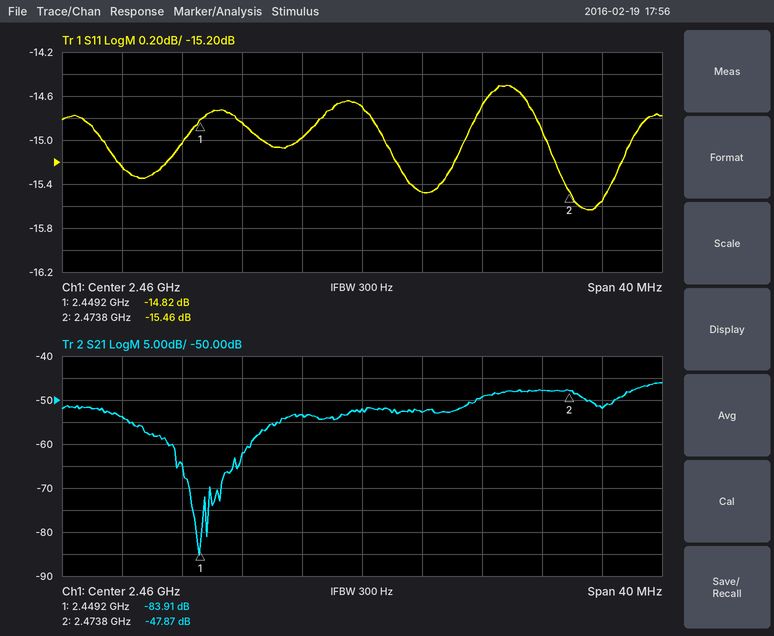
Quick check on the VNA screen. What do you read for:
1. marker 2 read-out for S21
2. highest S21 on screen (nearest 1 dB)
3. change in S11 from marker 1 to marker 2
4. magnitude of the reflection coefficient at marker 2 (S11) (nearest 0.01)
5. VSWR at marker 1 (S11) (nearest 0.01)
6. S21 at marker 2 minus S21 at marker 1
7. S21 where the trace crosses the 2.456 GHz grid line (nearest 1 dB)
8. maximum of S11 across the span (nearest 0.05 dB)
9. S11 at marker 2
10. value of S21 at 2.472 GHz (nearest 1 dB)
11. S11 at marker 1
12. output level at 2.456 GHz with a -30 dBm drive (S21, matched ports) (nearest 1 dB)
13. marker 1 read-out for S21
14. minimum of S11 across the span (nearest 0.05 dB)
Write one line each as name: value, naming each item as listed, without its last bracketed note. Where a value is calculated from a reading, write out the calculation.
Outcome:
marker 2 read-out for S21: -47.87 dB
highest S21 on screen: -46 dB
change in S11 from marker 1 to marker 2: -15.46 − (-14.82) = -0.64 dB
magnitude of the reflection coefficient at marker 2 (S11): 10^(-15.46/20) ≈ 0.17
VSWR at marker 1 (S11): (1 + 0.1816)/(1 − 0.1816) ≈ 1.44
S21 at marker 2 minus S21 at marker 1: -47.87 − (-83.91) = 36.04 dB
S21 where the trace crosses the 2.456 GHz grid line: -53 dB
maximum of S11 across the span: -14.50 dB
S11 at marker 2: -15.46 dB
value of S21 at 2.472 GHz: -48 dB
S11 at marker 1: -14.82 dB
output level at 2.456 GHz with a -30 dBm drive (S21, matched ports): -30 dBm + (-53 dB) = -83 dBm
marker 1 read-out for S21: -83.91 dB
minimum of S11 across the span: -15.65 dB
